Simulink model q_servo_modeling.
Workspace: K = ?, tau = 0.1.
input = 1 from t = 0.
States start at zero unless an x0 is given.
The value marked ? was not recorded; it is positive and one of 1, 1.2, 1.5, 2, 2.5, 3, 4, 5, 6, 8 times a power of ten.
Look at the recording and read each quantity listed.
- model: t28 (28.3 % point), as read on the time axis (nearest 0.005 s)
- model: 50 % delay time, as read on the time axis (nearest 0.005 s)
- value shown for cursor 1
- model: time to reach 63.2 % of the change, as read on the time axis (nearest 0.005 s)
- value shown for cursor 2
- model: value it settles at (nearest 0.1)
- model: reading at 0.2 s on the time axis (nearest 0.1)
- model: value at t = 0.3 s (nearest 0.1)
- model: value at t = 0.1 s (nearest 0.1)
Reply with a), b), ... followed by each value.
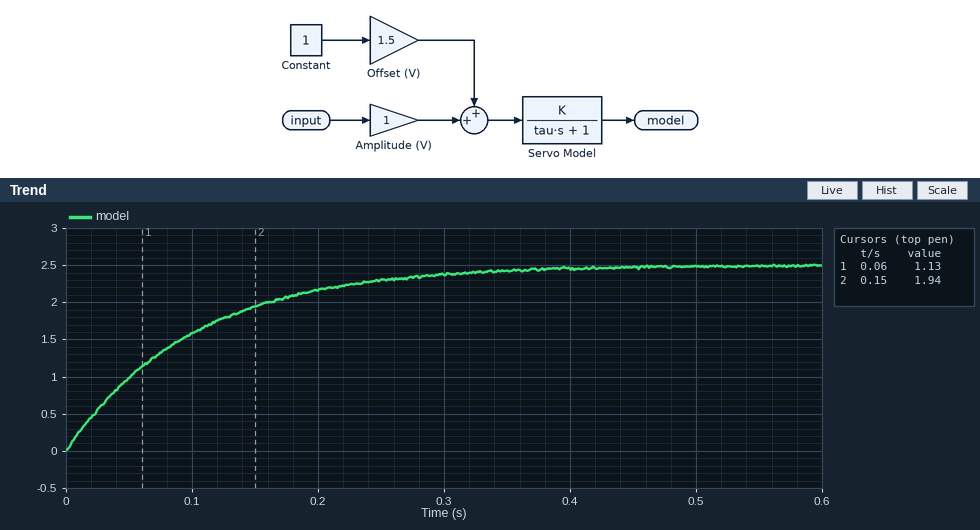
a) 0.035 s
b) 0.070 s
c) 1.13
d) 0.100 s
e) 1.94
f) 2.5
g) 2.2
h) 2.4
i) 1.6
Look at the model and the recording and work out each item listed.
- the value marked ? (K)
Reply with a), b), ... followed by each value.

a) 1
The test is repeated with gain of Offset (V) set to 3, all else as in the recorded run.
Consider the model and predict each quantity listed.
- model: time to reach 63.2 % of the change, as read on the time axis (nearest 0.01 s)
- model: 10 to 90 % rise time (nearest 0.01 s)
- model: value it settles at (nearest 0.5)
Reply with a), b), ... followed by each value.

a) 0.10 s
b) 0.22 s
c) 4.0
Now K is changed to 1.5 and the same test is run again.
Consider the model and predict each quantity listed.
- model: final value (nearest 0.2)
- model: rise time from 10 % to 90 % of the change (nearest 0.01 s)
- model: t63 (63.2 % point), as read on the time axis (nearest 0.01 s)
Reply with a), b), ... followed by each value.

a) 3.8
b) 0.22 s
c) 0.10 s
